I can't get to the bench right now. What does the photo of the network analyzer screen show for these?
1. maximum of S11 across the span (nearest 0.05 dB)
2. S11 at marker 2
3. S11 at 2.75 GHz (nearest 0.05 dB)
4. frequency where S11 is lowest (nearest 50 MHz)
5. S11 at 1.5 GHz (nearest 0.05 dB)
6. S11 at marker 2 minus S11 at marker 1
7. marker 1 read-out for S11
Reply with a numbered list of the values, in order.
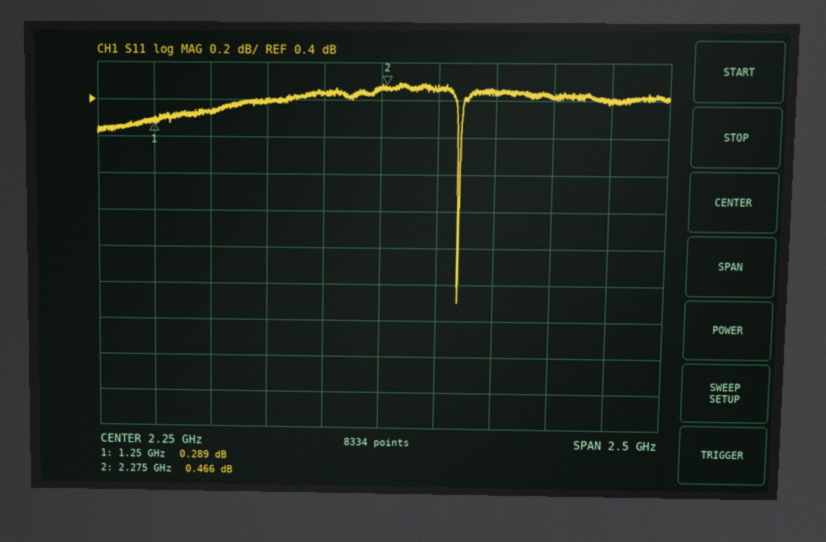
1. 0.50 dB
2. 0.466 dB
3. 0.45 dB
4. 2.60 GHz
5. 0.35 dB
6. 0.177 dB
7. 0.289 dB
